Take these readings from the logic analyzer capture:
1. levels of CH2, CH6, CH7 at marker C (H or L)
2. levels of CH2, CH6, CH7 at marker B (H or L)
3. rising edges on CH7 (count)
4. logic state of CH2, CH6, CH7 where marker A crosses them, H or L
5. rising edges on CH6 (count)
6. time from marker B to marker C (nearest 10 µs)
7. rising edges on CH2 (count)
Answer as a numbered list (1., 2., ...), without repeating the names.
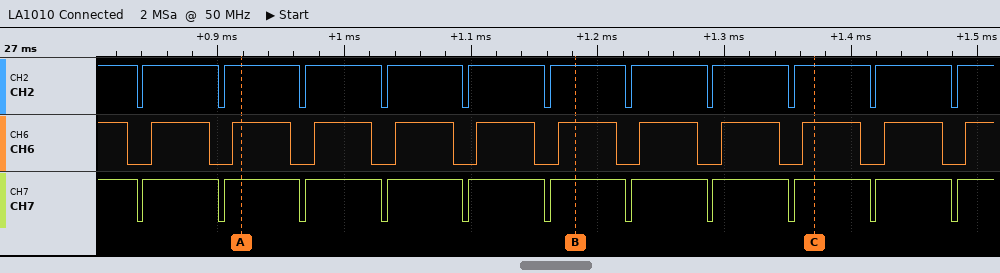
1. CH2=H, CH6=H, CH7=H
2. CH2=H, CH6=H, CH7=H
3. 11
4. CH2=H, CH6=H, CH7=H
5. 11
6. 190 µs
7. 11
